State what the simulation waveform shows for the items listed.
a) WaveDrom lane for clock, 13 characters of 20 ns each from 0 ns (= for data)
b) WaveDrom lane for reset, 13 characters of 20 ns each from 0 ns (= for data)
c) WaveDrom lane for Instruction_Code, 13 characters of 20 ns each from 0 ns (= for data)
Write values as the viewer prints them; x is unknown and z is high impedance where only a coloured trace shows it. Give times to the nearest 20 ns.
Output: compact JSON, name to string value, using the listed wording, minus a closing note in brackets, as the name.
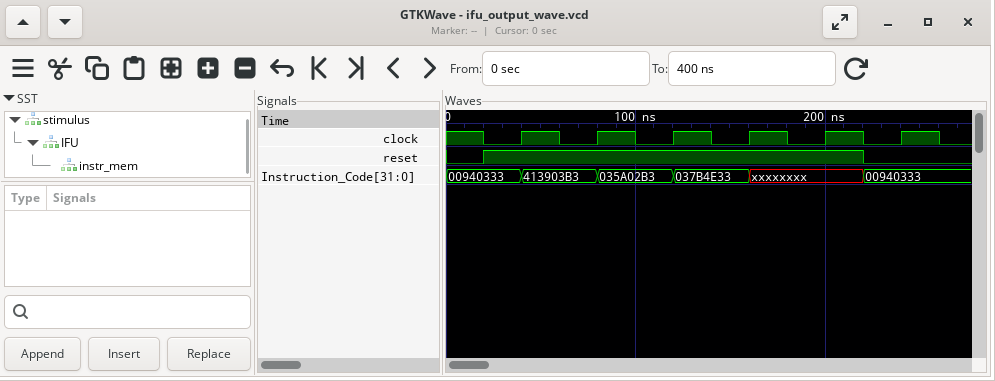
{"WaveDrom lane for clock, 13 characters of 20 ns each from 0 ns": "{name: 'clock', wave: '1010101010101'}", "WaveDrom lane for reset, 13 characters of 20 ns each from 0 ns": "{name: 'reset', wave: '01.........0.'}", "WaveDrom lane for Instruction_Code, 13 characters of 20 ns each from 0 ns": "{name: 'Instruction_Code', wave: '=.=.=.=.x..=.', data: '00940333 413903B3 035A02B3 037B4E33 00940333'}"}
